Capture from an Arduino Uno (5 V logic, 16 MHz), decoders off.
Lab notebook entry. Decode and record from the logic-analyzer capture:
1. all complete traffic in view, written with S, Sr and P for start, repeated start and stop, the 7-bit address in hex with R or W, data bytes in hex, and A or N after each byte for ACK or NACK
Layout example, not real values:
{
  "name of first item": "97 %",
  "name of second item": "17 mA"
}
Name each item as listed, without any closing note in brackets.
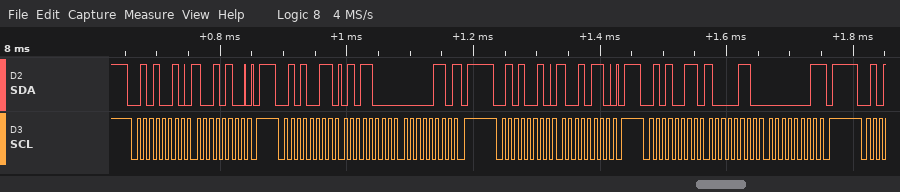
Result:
{
  "all complete traffic in view, written with S, Sr and P for start, repeated start and stop, the 7-bit address in hex with R or W, data bytes in hex, and A or N after each byte for ACK or NACK": "S 29W A 94 A P S 29R A 58 A 06 N P S 29W A 96 A P S 29R A 86 A 01 N P"
}
